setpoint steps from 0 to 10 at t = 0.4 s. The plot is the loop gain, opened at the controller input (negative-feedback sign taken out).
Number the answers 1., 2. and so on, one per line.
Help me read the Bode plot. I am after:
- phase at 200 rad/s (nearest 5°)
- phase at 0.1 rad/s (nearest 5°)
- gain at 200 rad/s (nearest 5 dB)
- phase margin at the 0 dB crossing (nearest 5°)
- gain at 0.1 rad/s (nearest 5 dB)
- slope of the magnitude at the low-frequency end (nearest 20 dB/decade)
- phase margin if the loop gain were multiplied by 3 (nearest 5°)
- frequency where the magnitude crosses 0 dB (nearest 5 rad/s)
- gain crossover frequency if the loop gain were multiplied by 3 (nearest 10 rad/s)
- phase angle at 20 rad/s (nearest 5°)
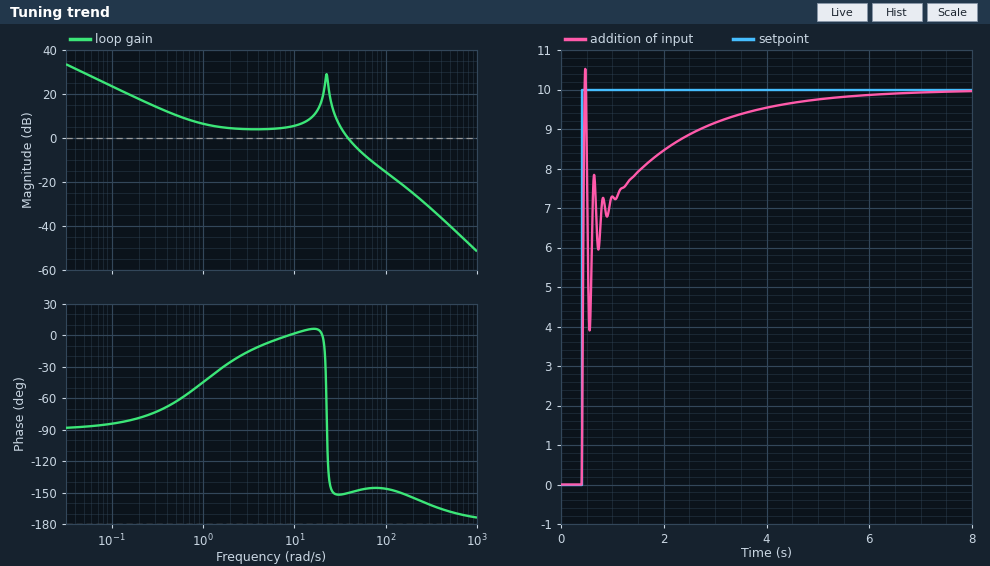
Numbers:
1. -155°
2. -85°
3. -25 dB
4. 30°
5. 25 dB
6. -20 dB/decade
7. 35°
8. 40 rad/s
9. 70 rad/s
10. 0°
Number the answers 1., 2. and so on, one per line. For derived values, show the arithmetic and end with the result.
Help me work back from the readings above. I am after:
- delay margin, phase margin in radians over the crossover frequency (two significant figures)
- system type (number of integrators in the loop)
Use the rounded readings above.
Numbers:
1. 30 × π / 180 / 40 = 0.013 s
2. 1
